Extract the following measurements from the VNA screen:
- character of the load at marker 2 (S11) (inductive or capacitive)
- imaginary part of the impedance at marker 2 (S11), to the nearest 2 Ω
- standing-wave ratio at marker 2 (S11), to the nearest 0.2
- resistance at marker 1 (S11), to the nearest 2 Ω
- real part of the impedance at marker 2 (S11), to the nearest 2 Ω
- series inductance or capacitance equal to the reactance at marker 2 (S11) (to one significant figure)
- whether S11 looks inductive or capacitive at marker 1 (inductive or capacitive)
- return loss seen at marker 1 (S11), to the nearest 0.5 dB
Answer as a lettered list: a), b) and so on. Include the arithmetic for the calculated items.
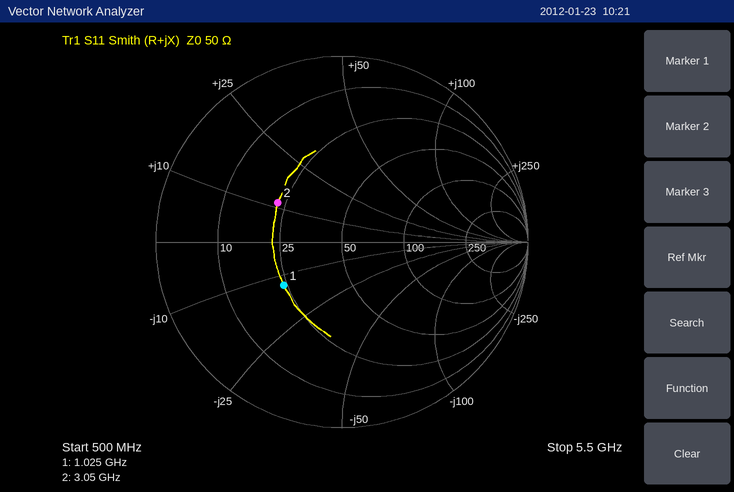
a) inductive
b) +12 Ω
c) 2.4
d) 24 Ω
e) 22 Ω
f) L = 12 Ω/(2π × 3.05 GHz) ≈ 626 pH, so 600 pH to one significant figure
g) capacitive
h) 8.0 dB
